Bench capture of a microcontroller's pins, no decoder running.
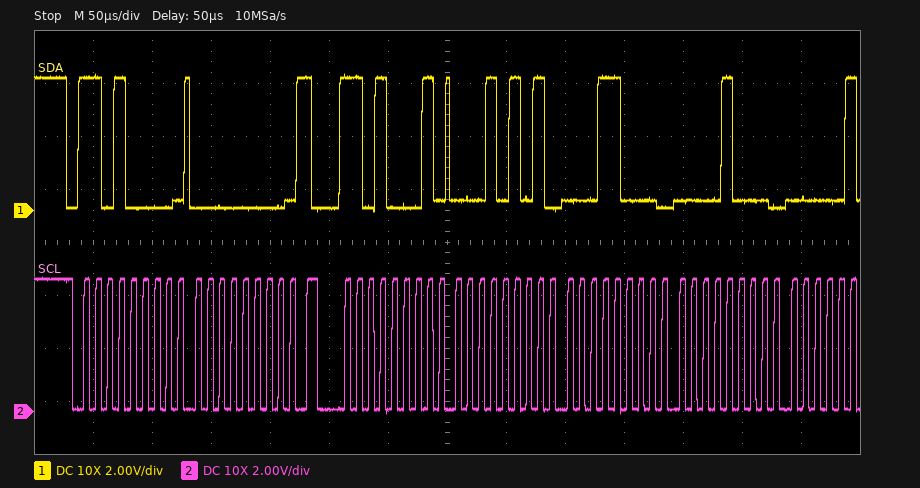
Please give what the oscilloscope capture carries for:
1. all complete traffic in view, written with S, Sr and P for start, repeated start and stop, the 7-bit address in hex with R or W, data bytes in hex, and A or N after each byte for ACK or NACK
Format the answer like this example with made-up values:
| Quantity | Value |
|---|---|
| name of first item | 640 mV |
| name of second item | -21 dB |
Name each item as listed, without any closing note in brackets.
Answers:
| Quantity | Value |
|---|---|
| all complete traffic in view, written with S, Sr and P for start, repeated start and stop, the 7-bit address in hex with R or W, data bytes in hex, and A or N after each byte for ACK or NACK | S 68W A 00 A Sr 68R A 15 A 18 A 08 A |
